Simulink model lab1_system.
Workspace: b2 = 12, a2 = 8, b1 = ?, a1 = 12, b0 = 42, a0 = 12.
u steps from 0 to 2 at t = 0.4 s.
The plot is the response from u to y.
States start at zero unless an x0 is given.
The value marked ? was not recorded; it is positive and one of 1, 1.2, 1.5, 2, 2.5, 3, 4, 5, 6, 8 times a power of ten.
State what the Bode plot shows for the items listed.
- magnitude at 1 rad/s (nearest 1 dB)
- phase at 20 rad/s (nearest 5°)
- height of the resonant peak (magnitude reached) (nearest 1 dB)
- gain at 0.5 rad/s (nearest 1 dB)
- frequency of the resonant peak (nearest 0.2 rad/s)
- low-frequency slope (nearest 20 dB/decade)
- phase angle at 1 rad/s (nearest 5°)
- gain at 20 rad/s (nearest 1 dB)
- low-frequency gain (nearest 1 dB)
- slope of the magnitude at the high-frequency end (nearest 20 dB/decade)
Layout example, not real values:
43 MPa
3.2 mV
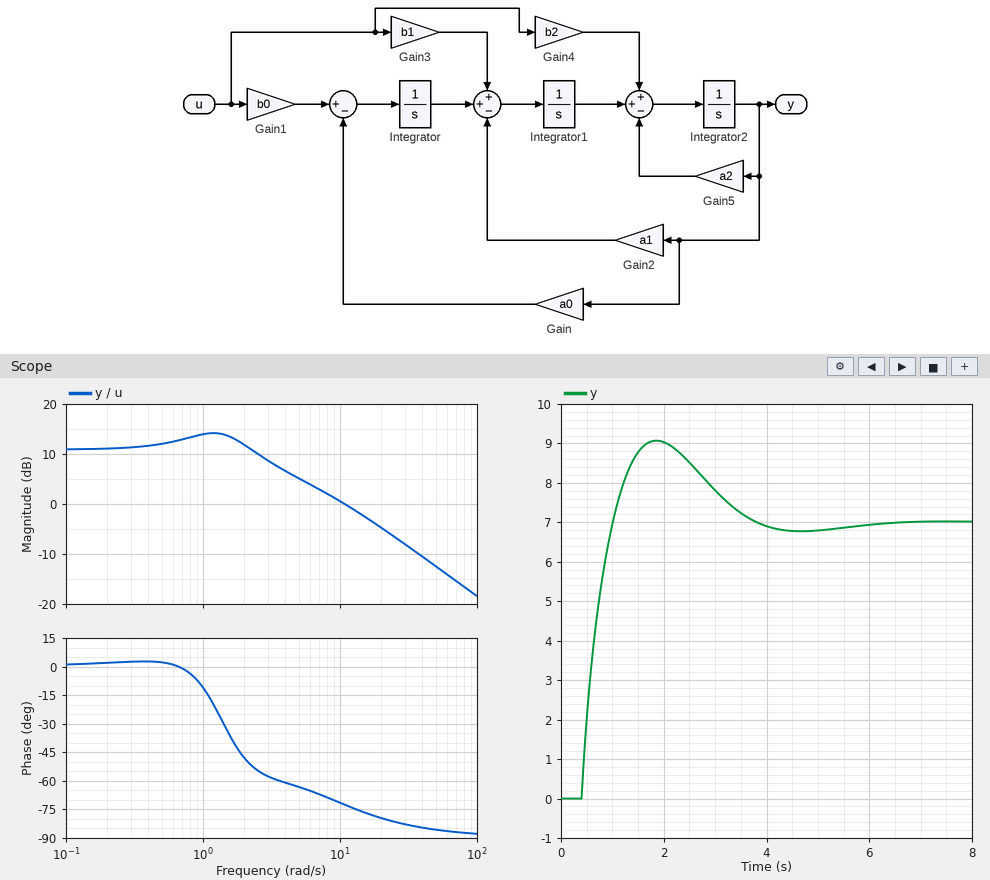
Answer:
14 dB
-80°
14 dB
12 dB
1.2 rad/s
0 dB/decade
-10°
-5 dB
11 dB
-20 dB/decade
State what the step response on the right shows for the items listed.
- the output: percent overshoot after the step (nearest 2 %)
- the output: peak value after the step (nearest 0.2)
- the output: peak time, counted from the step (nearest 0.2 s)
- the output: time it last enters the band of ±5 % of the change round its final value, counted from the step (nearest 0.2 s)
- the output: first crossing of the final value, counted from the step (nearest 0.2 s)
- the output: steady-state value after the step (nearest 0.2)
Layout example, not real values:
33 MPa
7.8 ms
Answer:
30 %
9.0
1.4 s
3.0 s
0.6 s
7.0
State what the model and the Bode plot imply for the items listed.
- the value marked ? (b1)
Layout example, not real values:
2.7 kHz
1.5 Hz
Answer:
50
